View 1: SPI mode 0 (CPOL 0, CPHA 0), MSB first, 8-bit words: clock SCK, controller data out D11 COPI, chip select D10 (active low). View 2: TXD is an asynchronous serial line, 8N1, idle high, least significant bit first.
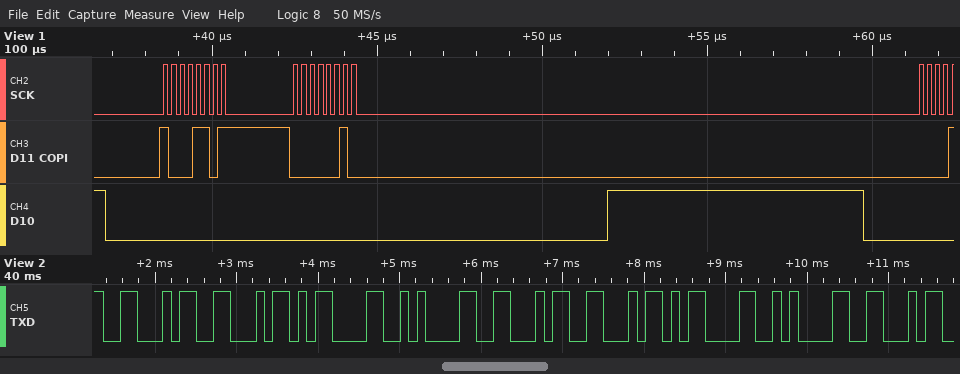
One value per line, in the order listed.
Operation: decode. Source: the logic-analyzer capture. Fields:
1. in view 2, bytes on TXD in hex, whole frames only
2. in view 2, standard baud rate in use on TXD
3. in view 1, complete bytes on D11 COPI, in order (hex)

46 46 0D 0A 46 46 0D 0A 46
9600 baud
8D 02
